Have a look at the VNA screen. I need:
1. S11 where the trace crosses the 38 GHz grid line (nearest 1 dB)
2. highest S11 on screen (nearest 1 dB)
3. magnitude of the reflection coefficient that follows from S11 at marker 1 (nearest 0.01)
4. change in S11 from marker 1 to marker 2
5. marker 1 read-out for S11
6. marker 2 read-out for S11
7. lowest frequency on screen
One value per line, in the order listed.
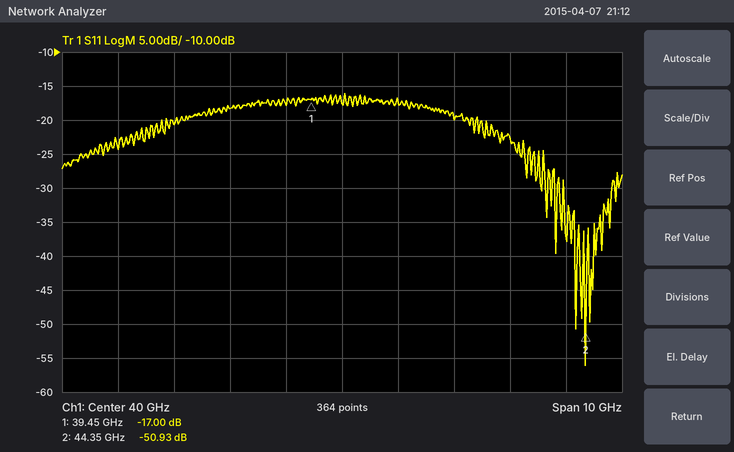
-18 dB
-16 dB
0.14
-33.93 dB
-17.00 dB
-50.93 dB
35 GHz
